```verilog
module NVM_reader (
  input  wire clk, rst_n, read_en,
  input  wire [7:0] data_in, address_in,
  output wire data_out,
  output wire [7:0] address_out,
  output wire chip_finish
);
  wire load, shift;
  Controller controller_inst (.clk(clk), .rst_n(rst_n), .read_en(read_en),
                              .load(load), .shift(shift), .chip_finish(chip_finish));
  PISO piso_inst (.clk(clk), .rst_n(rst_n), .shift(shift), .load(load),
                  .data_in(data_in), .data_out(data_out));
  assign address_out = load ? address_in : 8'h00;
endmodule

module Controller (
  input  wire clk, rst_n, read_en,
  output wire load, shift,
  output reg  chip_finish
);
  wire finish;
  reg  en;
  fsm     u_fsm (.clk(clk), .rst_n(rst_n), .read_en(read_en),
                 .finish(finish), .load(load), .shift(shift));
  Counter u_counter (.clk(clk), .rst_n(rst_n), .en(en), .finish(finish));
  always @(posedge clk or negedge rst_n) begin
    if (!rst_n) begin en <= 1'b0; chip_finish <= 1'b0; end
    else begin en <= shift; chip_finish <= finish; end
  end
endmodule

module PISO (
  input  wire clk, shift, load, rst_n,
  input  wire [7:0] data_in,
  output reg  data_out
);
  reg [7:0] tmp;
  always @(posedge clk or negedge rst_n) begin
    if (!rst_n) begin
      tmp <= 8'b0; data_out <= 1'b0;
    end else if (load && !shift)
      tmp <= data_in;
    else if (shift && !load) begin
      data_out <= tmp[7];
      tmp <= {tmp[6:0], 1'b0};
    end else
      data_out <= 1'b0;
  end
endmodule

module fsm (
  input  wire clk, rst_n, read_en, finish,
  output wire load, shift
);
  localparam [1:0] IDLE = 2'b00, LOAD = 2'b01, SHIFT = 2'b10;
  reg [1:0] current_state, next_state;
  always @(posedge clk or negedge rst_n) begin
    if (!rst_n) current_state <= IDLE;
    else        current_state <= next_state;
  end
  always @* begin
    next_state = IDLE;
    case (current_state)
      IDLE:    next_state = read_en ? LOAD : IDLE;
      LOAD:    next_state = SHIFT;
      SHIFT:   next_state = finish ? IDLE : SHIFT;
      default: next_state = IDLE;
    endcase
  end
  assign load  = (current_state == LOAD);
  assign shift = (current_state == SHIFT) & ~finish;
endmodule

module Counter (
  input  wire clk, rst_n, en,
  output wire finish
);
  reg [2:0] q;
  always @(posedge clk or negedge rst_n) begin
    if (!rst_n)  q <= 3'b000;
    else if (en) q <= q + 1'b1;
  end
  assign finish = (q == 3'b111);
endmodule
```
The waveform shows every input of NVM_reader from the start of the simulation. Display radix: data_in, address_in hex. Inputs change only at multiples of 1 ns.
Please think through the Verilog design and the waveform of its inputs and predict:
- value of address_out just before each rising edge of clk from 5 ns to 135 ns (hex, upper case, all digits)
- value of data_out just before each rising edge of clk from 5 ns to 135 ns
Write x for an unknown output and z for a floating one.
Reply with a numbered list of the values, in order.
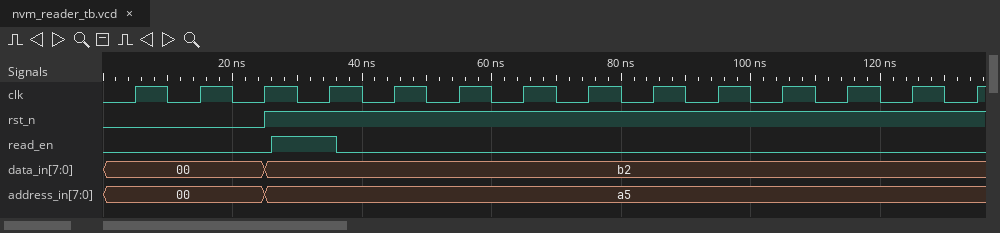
1. 00, 00, 00, 00, A5, 00, 00, 00, 00, 00, 00, 00, 00, 00
2. 0 0 0 0 0 0 1 0 1 1 0 0 1 0
